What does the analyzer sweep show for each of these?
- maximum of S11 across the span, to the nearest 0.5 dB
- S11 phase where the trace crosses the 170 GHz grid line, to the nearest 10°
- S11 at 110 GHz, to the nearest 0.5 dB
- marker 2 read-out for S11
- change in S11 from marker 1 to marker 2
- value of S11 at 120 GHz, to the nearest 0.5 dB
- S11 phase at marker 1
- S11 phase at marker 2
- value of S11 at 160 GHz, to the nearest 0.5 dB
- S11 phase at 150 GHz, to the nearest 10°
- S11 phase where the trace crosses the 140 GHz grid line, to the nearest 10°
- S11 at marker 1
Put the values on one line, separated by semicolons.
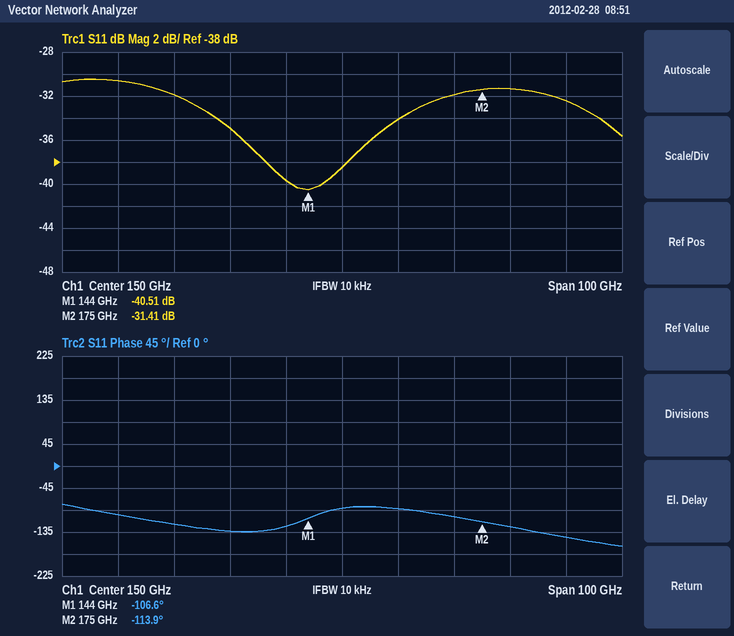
-30.5 dB; -100°; -30.5 dB; -31.41 dB; 9.10 dB; -32.0 dB; -106.6°; -113.9°; -34.0 dB; -90°; -120°; -40.51 dB
